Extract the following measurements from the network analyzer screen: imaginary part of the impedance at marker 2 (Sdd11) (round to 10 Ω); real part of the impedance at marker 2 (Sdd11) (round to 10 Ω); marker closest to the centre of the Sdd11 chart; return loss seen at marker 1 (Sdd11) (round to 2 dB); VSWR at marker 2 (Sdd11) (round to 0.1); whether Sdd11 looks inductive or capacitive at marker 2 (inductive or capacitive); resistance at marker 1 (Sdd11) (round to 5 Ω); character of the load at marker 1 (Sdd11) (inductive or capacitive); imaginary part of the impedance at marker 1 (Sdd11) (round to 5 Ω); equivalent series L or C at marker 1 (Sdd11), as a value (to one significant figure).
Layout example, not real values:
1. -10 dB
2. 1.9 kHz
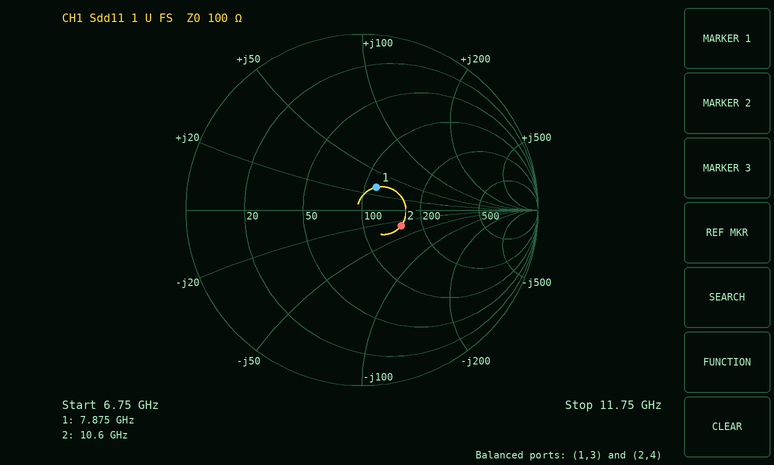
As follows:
1. -30 Ω
2. 150 Ω
3. marker 1
4. 16 dB
5. 1.6
6. capacitive
7. 115 Ω
8. inductive
9. +30 Ω
10. 600 pH
